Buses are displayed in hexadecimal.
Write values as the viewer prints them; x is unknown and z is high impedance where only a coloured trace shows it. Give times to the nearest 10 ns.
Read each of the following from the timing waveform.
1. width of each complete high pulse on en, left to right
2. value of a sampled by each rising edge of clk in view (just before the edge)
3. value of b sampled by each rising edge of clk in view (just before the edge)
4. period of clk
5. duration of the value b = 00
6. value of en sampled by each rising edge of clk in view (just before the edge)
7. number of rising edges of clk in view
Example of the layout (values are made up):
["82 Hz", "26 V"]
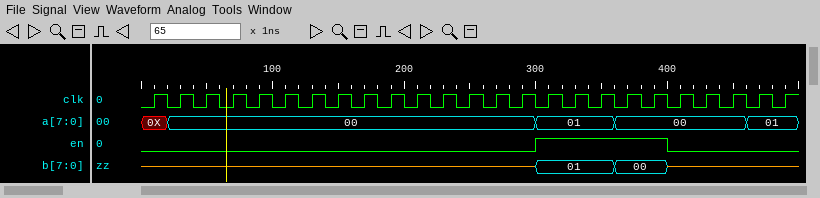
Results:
["100 ns", "0X, 00, 00, 00, 00, 00, 00, 00, 00, 00, 00, 00, 00, 00, 00, 01, 01, 01, 00, 00, 00, 00, 00, 01, 01", "z, z, z, z, z, z, z, z, z, z, z, z, z, z, z, 01, 01, 01, 00, 00, z, z, z, z, z", "20 ns", "40 ns", "0 0 0 0 0 0 0 0 0 0 0 0 0 0 0 1 1 1 1 1 0 0 0 0 0", "25"]
